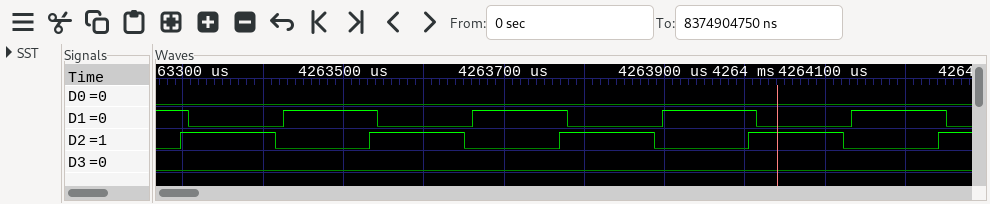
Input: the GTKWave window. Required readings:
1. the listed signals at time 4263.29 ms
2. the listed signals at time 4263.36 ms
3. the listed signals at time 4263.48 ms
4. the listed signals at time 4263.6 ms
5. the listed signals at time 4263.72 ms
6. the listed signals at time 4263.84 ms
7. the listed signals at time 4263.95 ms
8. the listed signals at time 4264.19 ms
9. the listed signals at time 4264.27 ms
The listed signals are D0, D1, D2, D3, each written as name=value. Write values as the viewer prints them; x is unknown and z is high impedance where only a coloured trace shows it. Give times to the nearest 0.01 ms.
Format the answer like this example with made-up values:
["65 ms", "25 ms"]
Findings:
["D0=0, D1=1, D2=0, D3=0", "D0=0, D1=0, D2=1, D3=0", "D0=0, D1=1, D2=0, D3=0", "D0=0, D1=0, D2=1, D3=0", "D0=0, D1=1, D2=0, D3=0", "D0=0, D1=0, D2=1, D3=0", "D0=0, D1=1, D2=0, D3=0", "D0=0, D1=1, D2=0, D3=0", "D0=0, D1=0, D2=1, D3=0"]
